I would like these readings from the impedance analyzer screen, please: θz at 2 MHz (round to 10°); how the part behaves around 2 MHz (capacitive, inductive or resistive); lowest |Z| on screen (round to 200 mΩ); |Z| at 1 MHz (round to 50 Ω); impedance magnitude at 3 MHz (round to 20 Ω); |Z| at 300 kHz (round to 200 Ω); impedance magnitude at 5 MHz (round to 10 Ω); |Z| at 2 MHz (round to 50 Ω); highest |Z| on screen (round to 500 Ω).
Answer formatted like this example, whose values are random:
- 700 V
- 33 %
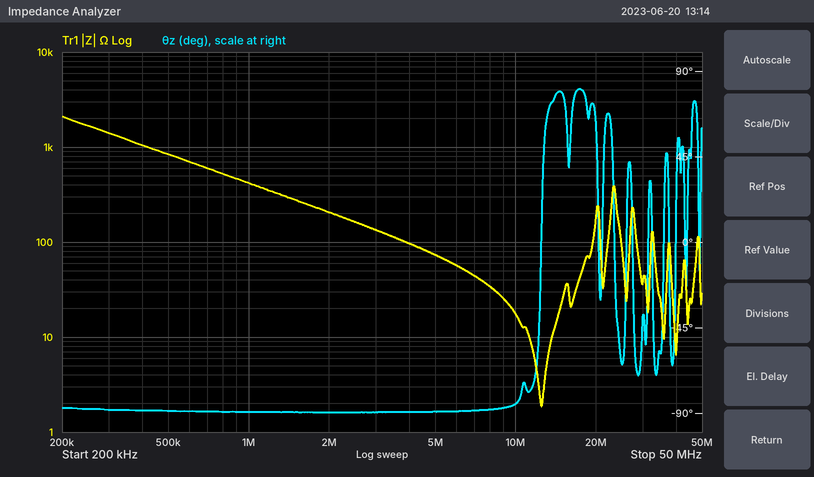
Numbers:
- -90°
- capacitive
- 1.8 Ω
- 400 Ω
- 140 Ω
- 1.4 kΩ
- 70 Ω
- 200 Ω
- 2.0 kΩ
